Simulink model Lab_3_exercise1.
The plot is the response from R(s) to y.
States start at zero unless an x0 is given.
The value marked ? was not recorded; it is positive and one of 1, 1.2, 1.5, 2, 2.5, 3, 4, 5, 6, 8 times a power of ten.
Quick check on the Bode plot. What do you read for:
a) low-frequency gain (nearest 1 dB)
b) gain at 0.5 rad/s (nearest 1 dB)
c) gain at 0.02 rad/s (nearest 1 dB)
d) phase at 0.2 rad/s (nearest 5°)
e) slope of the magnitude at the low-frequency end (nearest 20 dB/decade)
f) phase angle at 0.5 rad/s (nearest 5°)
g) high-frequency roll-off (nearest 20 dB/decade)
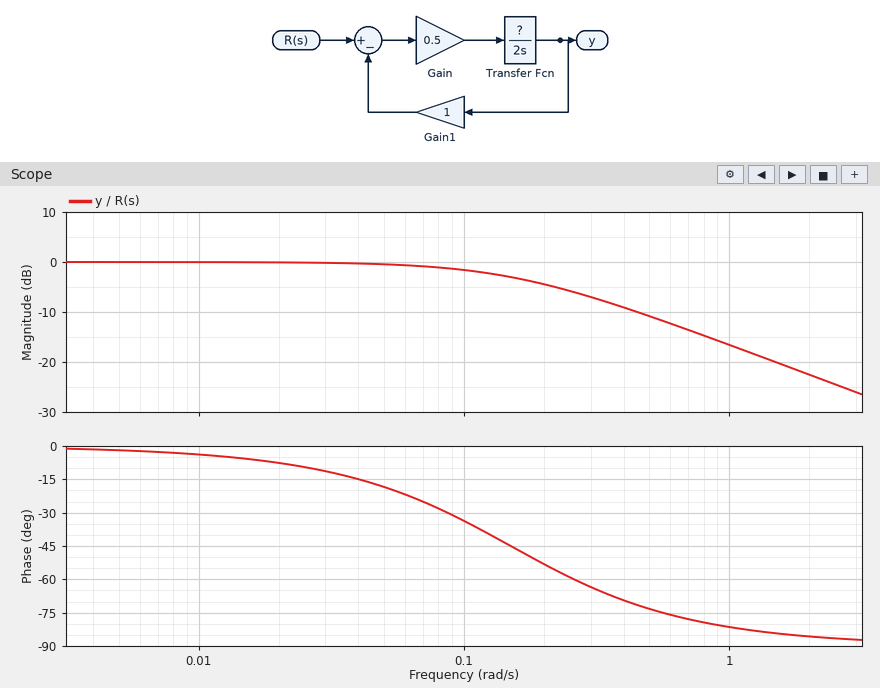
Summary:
0 dB
-11 dB
0 dB
-55°
0 dB/decade
-75°
-20 dB/decade
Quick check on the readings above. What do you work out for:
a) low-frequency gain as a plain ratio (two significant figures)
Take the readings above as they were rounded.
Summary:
1.0
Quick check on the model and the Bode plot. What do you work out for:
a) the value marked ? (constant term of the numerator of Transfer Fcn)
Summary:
0.6
